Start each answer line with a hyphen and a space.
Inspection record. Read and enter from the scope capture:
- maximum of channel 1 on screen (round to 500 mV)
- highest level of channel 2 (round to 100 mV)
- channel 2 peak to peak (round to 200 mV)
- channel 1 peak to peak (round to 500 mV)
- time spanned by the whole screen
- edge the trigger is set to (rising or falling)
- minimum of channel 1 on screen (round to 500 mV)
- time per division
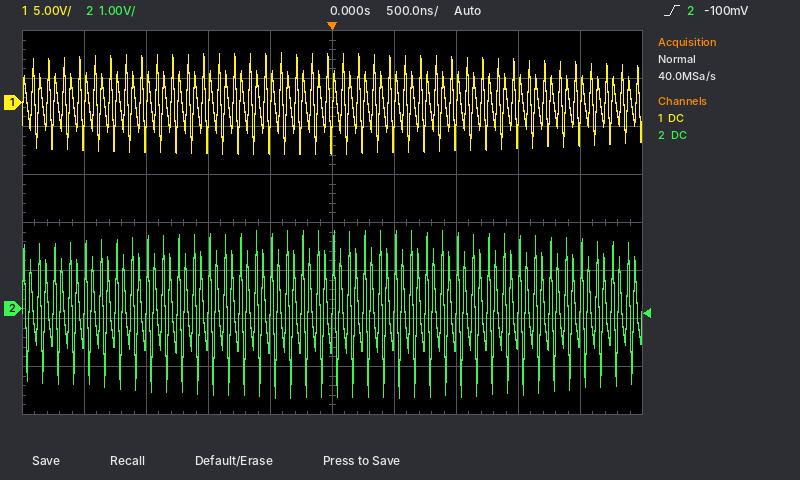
- 5.0 V
- 1.6 V
- 3.4 V
- 10.5 V
- 5 µs
- rising
- -5.5 V
- 500 ns
